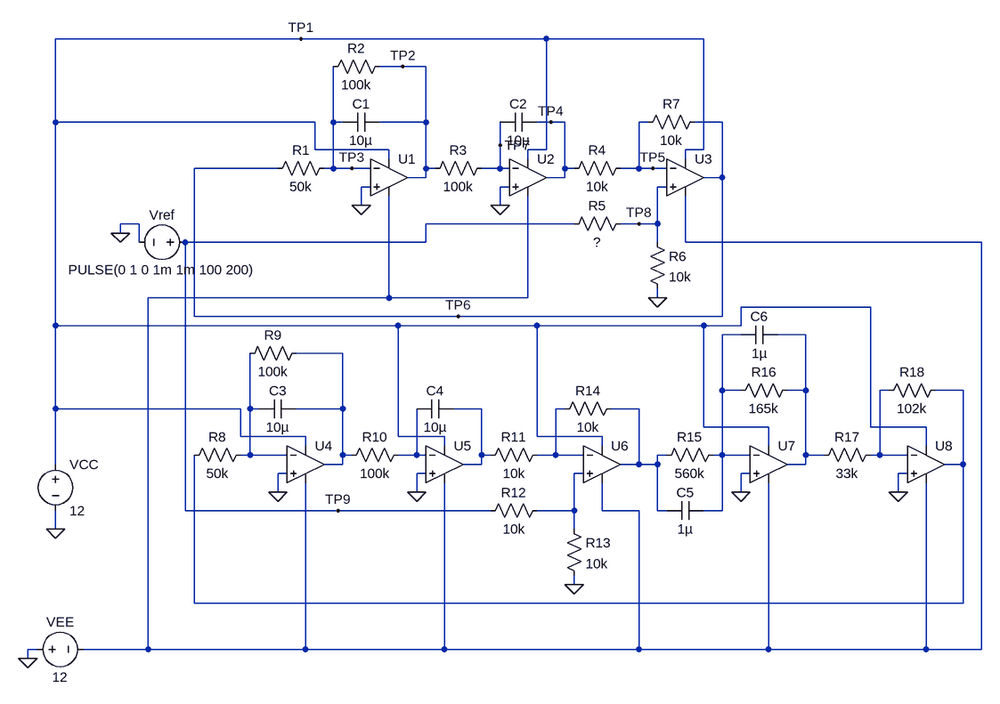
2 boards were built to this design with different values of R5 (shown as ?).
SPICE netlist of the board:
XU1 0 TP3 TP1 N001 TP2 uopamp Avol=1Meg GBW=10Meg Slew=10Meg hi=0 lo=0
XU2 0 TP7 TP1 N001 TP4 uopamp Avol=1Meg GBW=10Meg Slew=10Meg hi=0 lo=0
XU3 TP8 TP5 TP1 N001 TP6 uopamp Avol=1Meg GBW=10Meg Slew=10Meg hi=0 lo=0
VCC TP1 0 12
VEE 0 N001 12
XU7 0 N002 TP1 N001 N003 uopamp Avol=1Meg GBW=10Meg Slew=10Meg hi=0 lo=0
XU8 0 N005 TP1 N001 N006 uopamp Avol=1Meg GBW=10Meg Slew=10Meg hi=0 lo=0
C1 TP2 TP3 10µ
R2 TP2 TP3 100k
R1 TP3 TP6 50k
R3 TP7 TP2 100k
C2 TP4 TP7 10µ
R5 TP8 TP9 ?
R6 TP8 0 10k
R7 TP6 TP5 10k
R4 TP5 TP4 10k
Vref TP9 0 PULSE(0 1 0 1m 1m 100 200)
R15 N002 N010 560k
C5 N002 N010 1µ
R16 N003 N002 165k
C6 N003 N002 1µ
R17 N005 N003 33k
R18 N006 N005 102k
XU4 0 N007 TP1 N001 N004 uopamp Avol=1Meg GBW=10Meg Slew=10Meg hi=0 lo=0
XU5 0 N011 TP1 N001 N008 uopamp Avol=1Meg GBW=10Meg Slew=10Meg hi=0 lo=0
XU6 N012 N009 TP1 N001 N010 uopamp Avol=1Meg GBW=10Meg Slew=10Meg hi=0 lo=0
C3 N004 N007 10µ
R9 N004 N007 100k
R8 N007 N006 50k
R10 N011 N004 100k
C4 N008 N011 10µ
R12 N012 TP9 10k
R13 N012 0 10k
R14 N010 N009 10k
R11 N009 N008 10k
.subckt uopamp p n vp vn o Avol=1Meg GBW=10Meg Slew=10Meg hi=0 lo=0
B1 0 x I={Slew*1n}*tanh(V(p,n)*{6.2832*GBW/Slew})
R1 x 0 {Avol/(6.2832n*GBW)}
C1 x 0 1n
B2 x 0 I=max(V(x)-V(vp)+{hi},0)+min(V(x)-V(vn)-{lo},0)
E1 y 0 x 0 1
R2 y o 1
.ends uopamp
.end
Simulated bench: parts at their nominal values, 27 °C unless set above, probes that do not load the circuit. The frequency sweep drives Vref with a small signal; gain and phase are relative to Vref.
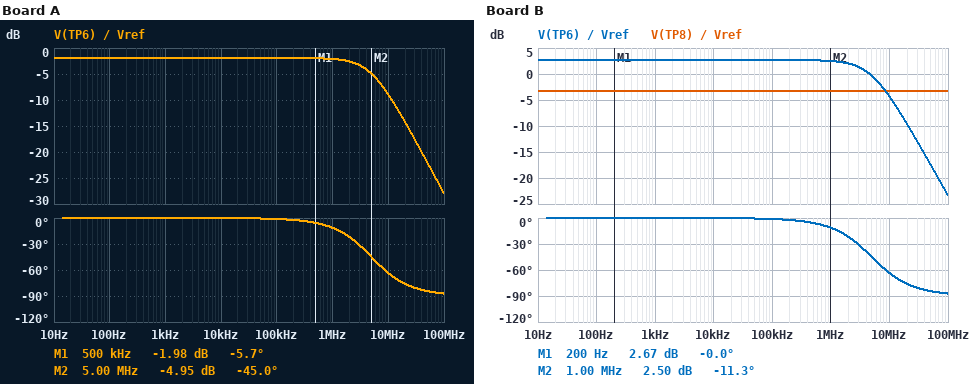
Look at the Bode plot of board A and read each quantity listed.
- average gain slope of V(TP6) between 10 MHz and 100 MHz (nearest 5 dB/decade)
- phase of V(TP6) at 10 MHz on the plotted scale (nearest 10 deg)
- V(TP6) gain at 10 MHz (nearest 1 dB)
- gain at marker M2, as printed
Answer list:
-20 dB/decade
-60 deg
-9 dB
-4.95 dB
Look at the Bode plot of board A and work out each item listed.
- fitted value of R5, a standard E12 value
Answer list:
15 kΩ
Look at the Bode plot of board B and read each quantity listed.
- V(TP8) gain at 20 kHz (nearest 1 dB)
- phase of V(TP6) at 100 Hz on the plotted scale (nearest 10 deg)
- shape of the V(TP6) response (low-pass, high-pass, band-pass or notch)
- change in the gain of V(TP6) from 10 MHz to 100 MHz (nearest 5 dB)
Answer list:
-3 dB
0 deg
low-pass
-20 dB
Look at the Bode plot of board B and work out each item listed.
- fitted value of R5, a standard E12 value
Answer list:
4.7 kΩ
